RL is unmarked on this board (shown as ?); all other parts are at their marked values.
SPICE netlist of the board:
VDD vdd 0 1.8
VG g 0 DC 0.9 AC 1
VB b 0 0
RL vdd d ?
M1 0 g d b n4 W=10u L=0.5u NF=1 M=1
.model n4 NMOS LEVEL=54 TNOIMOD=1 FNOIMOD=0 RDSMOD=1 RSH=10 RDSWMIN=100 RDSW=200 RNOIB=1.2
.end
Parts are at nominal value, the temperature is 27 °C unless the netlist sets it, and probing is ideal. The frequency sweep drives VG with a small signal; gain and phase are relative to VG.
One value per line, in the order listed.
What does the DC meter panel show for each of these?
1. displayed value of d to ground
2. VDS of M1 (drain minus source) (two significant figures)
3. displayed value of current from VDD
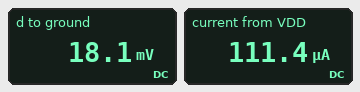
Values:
18.1 mV
-18 mV
111.4 µA
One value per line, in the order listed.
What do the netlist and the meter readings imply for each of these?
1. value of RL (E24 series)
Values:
16 kΩ
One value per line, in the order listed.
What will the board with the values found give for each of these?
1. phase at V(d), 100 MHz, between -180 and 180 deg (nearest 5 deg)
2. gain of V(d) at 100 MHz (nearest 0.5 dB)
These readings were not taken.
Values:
170 deg
-32.5 dB
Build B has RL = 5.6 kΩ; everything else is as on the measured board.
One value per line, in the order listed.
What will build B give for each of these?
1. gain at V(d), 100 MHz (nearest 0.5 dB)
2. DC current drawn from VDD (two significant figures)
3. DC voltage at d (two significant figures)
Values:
-23.0 dB
310 µA
53 mV
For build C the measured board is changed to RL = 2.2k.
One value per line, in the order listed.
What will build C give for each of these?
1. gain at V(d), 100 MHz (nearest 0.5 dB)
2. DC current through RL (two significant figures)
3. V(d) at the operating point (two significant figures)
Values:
-12.5 dB
750 µA
140 mV
